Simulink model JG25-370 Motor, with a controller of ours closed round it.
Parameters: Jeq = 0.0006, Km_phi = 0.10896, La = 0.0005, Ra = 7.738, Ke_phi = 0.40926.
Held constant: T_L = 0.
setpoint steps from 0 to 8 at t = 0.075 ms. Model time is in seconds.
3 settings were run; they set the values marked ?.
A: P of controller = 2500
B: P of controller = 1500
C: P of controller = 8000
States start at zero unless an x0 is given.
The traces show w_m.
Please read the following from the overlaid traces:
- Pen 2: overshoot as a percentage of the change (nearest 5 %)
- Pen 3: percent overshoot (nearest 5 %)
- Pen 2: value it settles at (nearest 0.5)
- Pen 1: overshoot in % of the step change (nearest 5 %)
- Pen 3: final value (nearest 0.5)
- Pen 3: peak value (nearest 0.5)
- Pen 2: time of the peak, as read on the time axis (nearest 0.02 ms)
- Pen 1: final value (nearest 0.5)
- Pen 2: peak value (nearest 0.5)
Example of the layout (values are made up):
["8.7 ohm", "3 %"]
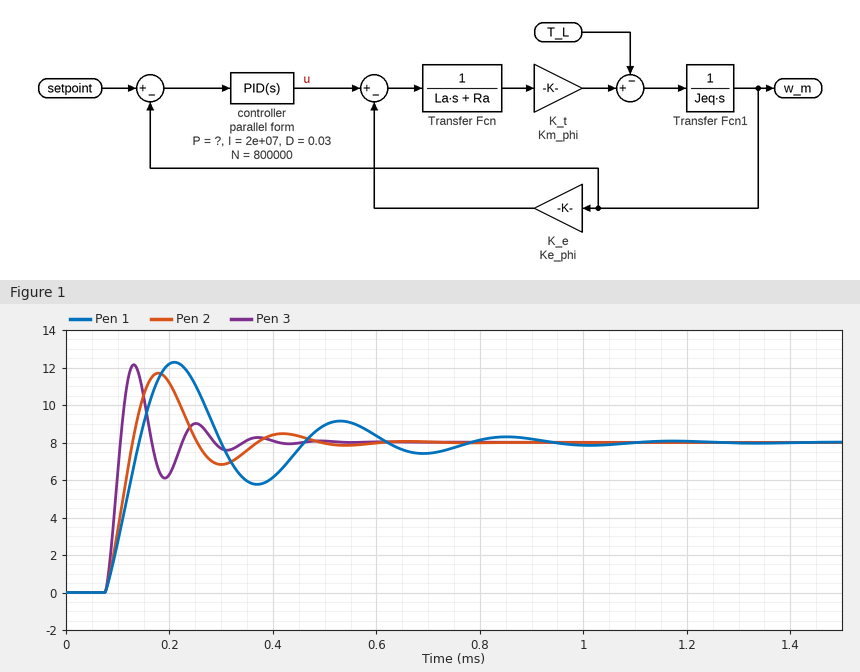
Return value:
["45 %", "50 %", "8.0", "55 %", "8.0", "12.0", "0.18 ms", "8.0", "11.5"]
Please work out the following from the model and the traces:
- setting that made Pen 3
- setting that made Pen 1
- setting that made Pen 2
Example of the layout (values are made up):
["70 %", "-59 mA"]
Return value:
["C", "B", "A"]
